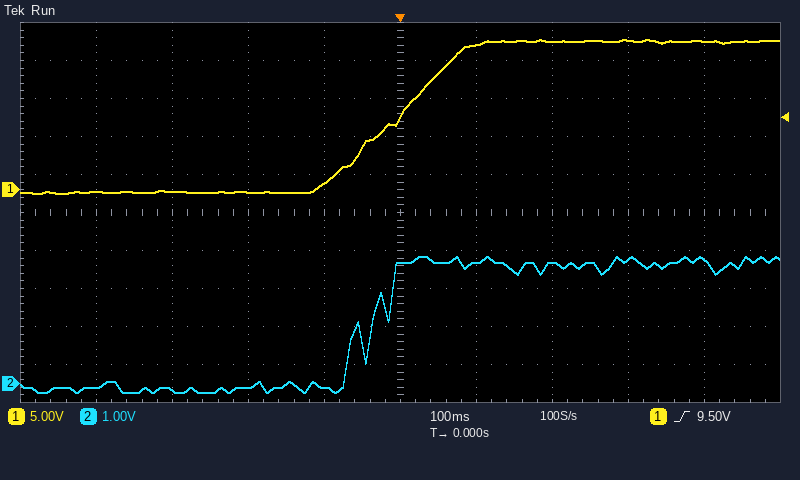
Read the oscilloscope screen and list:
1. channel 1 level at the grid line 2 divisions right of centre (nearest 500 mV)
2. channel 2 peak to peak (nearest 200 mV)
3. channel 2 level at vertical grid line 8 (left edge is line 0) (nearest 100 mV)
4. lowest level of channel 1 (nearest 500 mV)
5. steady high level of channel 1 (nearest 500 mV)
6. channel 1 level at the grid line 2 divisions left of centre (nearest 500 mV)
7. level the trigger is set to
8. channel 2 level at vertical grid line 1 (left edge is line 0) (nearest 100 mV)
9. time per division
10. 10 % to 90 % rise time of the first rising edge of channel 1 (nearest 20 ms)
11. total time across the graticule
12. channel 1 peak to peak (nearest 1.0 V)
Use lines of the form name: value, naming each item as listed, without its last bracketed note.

channel 1 level at the grid line 2 divisions right of centre: 19.5 V
channel 2 peak to peak: 3.6 V
channel 2 level at vertical grid line 8 (left edge is line 0): 3.3 V
lowest level of channel 1: -500 mV
steady high level of channel 1: 19.5 V
channel 1 level at the grid line 2 divisions left of centre: -500 mV
level the trigger is set to: 9.50 V
channel 2 level at vertical grid line 1 (left edge is line 0): -100 mV
time per division: 100 ms
10 % to 90 % rise time of the first rising edge of channel 1: 160 ms
total time across the graticule: 1 s
channel 1 peak to peak: 20.0 V
